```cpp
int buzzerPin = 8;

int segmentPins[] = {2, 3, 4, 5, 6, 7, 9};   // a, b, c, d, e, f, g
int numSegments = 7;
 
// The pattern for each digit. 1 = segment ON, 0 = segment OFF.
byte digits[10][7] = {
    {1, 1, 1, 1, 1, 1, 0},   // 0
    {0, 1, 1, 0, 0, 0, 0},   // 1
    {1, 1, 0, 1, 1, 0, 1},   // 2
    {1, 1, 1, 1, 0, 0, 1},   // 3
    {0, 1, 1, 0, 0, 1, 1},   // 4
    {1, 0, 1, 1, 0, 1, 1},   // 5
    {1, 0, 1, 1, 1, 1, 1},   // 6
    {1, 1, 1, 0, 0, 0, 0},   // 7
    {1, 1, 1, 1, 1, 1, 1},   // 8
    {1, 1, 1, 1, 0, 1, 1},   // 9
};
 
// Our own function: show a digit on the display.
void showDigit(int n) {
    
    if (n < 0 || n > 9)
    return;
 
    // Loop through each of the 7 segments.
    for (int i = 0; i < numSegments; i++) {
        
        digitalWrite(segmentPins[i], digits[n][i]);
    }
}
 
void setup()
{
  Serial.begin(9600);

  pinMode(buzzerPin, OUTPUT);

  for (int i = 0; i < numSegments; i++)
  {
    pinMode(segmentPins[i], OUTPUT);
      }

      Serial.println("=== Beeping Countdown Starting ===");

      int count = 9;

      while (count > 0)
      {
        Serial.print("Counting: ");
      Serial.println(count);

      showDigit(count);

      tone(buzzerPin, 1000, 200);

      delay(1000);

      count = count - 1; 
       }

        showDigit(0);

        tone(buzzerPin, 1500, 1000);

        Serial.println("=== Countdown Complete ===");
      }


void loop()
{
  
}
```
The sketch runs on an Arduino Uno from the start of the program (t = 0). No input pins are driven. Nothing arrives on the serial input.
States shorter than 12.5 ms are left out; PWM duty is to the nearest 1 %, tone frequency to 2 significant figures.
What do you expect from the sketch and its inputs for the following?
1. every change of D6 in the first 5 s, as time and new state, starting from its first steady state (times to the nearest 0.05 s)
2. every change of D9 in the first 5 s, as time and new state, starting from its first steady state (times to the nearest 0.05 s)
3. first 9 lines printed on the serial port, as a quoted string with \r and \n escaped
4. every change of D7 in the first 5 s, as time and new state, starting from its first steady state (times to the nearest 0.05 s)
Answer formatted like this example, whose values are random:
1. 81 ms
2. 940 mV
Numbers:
1. 0 s low; 1 s high; 2 s low; 3 s high; 4 s low
2. 0 s high; 2 s low; 3 s high
3. "=== Beeping Countdown Starting ===\r\nCounting: 9\r\nCounting: 8\r\nCounting: 7\r\nCounting: 6\r\nCounting: 5\r\nCounting: 4\r\nCounting: 3\r\nCounting: 2\r\n"
4. 0 s high; 2 s low; 3 s high
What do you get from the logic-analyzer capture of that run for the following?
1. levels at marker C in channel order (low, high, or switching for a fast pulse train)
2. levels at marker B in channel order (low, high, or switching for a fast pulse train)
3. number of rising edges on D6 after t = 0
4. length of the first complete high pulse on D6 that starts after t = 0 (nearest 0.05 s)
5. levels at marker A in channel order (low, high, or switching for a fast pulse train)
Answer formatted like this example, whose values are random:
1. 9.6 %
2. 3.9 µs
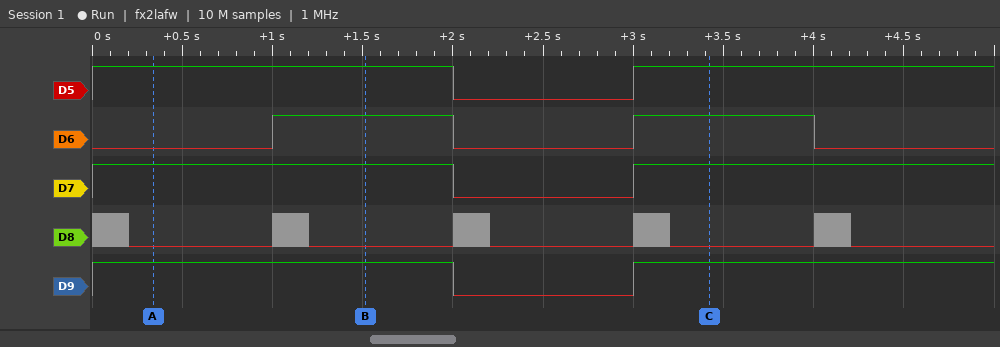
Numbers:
1. D5 high, D6 high, D7 high, D8 low, D9 high
2. D5 high, D6 high, D7 high, D8 low, D9 high
3. 2
4. 1.00 s
5. D5 high, D6 low, D7 high, D8 low, D9 high
